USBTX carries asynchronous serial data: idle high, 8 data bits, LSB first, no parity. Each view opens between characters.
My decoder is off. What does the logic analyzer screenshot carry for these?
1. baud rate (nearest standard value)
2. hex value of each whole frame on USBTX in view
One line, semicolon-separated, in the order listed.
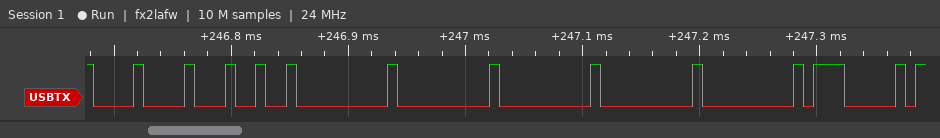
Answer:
115200 baud; 08, 24, 00, 00, 00, 00, 00, 07
